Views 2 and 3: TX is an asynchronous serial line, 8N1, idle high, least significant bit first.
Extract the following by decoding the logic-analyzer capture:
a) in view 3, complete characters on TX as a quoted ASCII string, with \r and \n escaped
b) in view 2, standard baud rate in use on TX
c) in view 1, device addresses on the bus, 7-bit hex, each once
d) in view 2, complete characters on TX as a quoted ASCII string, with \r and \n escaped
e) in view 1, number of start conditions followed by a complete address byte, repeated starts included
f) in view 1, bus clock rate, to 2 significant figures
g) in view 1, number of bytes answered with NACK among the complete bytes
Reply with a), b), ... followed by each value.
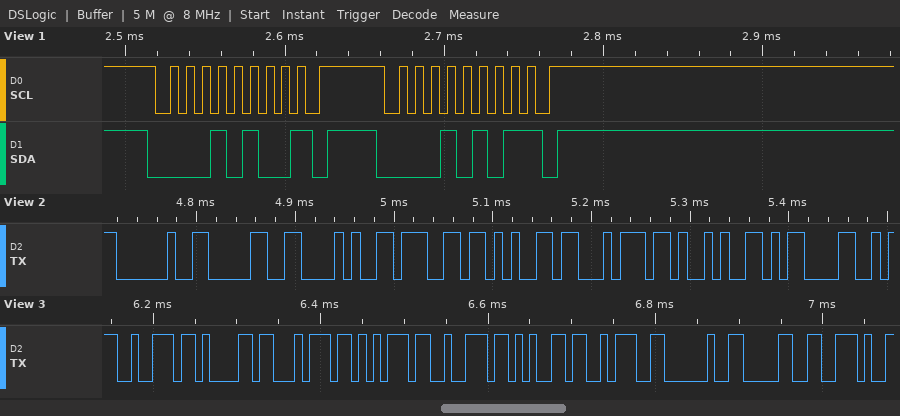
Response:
a) "rature: 0."
b) 115200 baud
c) 0x0A
d) " 0(get)\r"
e) 2
f) 100 kHz
g) 2
